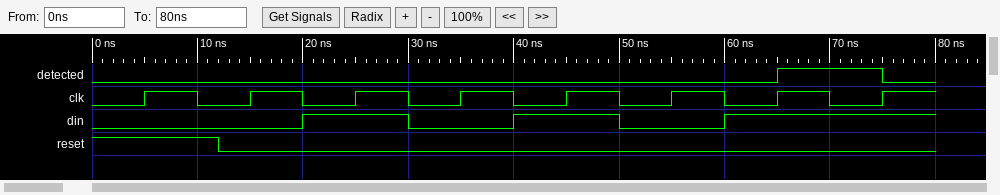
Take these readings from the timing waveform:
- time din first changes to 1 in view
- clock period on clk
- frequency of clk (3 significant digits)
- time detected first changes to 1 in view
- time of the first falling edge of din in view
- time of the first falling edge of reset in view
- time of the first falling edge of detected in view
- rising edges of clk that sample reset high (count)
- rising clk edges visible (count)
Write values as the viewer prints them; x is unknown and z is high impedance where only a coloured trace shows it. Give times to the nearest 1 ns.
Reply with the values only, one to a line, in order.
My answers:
20 ns
10 ns
100 MHz
65 ns
30 ns
12 ns
75 ns
1
8
